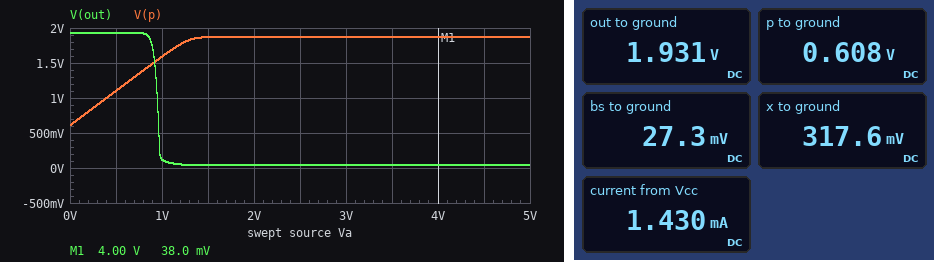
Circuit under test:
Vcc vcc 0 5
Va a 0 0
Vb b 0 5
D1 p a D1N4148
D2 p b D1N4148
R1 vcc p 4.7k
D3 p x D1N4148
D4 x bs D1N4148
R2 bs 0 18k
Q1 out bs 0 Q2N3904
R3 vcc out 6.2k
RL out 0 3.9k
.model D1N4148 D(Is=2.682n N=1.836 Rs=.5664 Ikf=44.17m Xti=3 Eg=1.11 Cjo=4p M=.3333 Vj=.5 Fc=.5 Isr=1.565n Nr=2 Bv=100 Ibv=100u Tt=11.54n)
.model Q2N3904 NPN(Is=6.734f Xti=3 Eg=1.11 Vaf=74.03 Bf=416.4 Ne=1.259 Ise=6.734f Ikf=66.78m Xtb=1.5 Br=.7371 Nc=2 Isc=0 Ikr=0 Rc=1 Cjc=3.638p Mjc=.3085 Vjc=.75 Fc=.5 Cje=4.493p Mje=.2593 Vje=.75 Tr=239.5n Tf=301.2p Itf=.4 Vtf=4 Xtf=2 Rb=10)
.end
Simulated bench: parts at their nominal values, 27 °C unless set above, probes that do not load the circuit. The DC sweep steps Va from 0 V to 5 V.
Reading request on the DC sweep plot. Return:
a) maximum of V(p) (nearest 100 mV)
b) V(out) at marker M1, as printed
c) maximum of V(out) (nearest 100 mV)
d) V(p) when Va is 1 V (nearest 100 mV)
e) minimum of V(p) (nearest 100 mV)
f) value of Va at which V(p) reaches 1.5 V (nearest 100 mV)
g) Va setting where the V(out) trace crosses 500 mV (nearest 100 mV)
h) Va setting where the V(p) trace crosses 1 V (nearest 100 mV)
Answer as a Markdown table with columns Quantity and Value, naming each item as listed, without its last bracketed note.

| Quantity | Value |
|---|---|
| maximum of V(p) | 1.9 V |
| V(out) at marker M1, as printed | 38.0 mV |
| maximum of V(out) | 1.9 V |
| V(p) when Va is 1 V | 1.6 V |
| minimum of V(p) | 600 mV |
| value of Va at which V(p) reaches 1.5 V | 900 mV |
| Va setting where the V(out) trace crosses 500 mV | 1.0 V |
| Va setting where the V(p) trace crosses 1 V | 400 mV |
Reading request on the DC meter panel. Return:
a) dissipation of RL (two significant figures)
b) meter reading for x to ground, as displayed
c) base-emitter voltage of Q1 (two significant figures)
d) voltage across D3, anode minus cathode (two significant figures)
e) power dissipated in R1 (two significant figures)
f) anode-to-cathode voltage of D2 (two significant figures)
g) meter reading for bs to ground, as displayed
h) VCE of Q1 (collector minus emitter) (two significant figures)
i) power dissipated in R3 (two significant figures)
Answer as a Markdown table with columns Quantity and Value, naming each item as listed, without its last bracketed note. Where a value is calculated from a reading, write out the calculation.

| Quantity | Value |
|---|---|
| dissipation of RL | (1.931 V)^2 / 3.9 kΩ = 960 µW |
| meter reading for x to ground, as displayed | 317.6 mV |
| base-emitter voltage of Q1 | 27.3 mV = 27 mV |
| voltage across D3, anode minus cathode | 608 mV - 317.6 mV = 290 mV |
| power dissipated in R1 | (5 V - 608 mV)^2 / 4.7 kΩ = 4.1 mW |
| anode-to-cathode voltage of D2 | 608 mV - 5 V = -4.4 V |
| meter reading for bs to ground, as displayed | 27.3 mV |
| VCE of Q1 (collector minus emitter) | 1.931 V = 1.9 V |
| power dissipated in R3 | (5 V - 1.931 V)^2 / 6.2 kΩ = 1.5 mW |
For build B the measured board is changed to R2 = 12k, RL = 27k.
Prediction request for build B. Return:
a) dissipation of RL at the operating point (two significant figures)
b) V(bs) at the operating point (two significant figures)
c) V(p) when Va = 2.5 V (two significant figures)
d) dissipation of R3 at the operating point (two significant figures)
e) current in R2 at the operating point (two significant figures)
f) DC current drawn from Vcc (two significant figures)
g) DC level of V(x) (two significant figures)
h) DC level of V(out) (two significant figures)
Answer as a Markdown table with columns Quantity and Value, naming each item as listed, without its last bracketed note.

| Quantity | Value |
|---|---|
| dissipation of RL at the operating point | 610 µW |
| V(bs) at the operating point | 20 mV |
| V(p) when Va = 2.5 V | 1.9 V |
| dissipation of R3 at the operating point | 140 µW |
| current in R2 at the operating point | 1.6 µA |
| DC current drawn from Vcc | 1.1 mA |
| DC level of V(x) | 310 mV |
| DC level of V(out) | 4.1 V |
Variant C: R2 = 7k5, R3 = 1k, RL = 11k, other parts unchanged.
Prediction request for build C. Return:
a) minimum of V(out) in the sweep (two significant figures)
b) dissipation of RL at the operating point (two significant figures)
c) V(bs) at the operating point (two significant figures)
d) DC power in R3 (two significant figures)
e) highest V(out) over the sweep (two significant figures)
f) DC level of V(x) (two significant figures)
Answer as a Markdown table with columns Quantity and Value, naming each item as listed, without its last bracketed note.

| Quantity | Value |
|---|---|
| minimum of V(out) in the sweep | 77 mV |
| dissipation of RL at the operating point | 1.9 mW |
| V(bs) at the operating point | 13 mV |
| DC power in R3 | 170 µW |
| highest V(out) over the sweep | 4.6 V |
| DC level of V(x) | 310 mV |
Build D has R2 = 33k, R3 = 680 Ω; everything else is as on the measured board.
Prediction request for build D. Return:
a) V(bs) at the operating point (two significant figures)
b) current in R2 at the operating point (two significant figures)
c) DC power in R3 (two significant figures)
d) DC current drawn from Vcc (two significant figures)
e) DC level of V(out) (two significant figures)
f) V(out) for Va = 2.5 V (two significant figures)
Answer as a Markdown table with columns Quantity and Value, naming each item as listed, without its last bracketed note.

| Quantity | Value |
|---|---|
| V(bs) at the operating point | 43 mV |
| current in R2 at the operating point | 1.3 µA |
| DC power in R3 | 810 µW |
| DC current drawn from Vcc | 2.0 mA |
| DC level of V(out) | 4.3 V |
| V(out) for Va = 2.5 V | 87 mV |
